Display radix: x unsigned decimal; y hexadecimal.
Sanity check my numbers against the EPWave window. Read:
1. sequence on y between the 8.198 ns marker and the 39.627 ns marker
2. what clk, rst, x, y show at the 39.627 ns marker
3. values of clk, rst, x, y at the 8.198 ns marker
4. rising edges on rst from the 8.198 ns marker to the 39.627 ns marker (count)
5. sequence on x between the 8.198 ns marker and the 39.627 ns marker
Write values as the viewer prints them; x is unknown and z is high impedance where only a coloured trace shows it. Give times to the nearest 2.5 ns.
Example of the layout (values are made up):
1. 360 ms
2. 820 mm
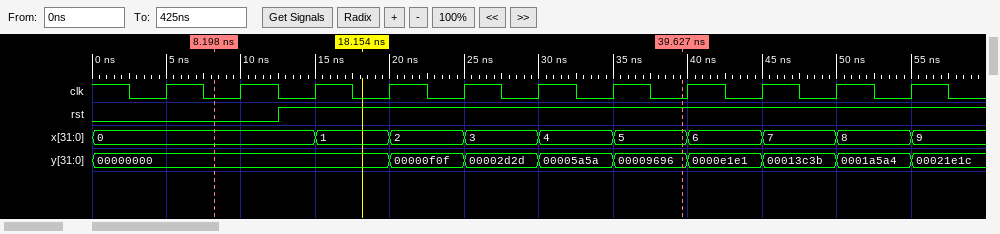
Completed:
1. 00000000, 00000f0f, 00002d2d, 00005a5a, 00009696
2. clk=0, rst=1, x=5, y=00009696
3. clk=0, rst=0, x=0, y=00000000
4. 1
5. 0, 1, 2, 3, 4, 5
